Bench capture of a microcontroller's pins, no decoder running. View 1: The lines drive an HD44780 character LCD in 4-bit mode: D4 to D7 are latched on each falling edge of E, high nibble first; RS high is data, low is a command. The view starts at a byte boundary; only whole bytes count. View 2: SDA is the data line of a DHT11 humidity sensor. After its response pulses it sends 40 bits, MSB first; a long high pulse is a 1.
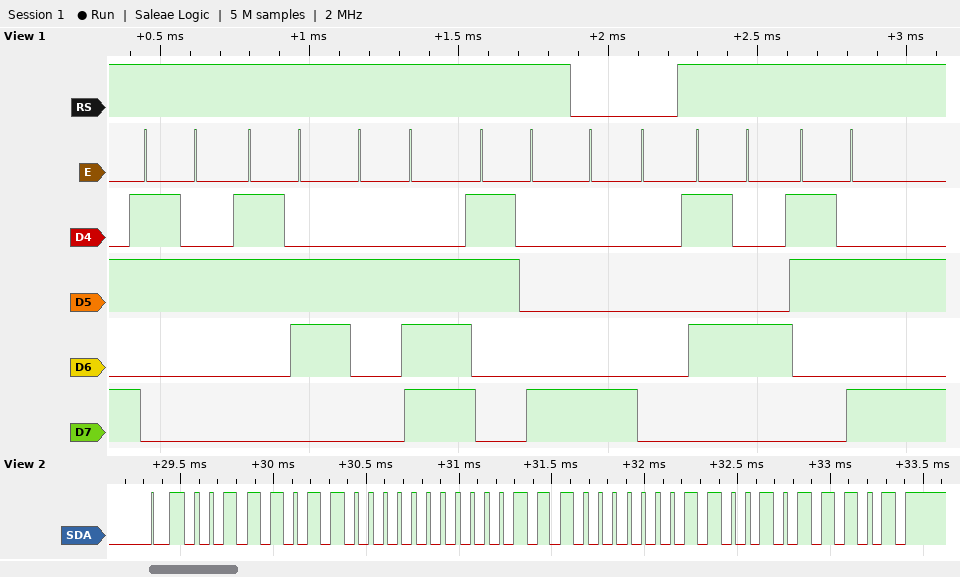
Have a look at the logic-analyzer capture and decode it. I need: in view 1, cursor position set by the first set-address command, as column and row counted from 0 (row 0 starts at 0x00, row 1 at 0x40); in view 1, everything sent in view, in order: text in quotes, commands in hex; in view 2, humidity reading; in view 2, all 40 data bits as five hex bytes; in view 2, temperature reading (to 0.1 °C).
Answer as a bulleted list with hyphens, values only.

- column 0, row 0
- "26.8" 0x80 "T:"
- 59 %
- 3B 00 1C 06 5D
- 28.6 °C
